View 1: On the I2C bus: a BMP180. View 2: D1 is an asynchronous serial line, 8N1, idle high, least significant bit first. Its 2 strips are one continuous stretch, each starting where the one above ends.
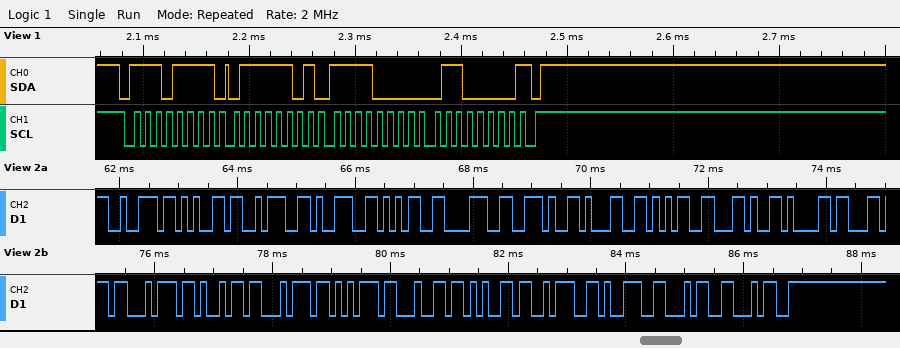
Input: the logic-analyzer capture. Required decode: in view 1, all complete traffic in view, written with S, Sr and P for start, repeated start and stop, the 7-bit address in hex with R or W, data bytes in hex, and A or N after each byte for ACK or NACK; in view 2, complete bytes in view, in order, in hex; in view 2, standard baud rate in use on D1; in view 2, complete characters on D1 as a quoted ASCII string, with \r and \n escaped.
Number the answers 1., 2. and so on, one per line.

1. S 77R A 7D A F0 A 60 N P
2. 72 65 3A 39 35 38 2E 31 35 2C 61 6C 74 69 74 75 64 65 3A 39 34 34
3. 9600 baud
4. "re:958.15,altitude:944"
